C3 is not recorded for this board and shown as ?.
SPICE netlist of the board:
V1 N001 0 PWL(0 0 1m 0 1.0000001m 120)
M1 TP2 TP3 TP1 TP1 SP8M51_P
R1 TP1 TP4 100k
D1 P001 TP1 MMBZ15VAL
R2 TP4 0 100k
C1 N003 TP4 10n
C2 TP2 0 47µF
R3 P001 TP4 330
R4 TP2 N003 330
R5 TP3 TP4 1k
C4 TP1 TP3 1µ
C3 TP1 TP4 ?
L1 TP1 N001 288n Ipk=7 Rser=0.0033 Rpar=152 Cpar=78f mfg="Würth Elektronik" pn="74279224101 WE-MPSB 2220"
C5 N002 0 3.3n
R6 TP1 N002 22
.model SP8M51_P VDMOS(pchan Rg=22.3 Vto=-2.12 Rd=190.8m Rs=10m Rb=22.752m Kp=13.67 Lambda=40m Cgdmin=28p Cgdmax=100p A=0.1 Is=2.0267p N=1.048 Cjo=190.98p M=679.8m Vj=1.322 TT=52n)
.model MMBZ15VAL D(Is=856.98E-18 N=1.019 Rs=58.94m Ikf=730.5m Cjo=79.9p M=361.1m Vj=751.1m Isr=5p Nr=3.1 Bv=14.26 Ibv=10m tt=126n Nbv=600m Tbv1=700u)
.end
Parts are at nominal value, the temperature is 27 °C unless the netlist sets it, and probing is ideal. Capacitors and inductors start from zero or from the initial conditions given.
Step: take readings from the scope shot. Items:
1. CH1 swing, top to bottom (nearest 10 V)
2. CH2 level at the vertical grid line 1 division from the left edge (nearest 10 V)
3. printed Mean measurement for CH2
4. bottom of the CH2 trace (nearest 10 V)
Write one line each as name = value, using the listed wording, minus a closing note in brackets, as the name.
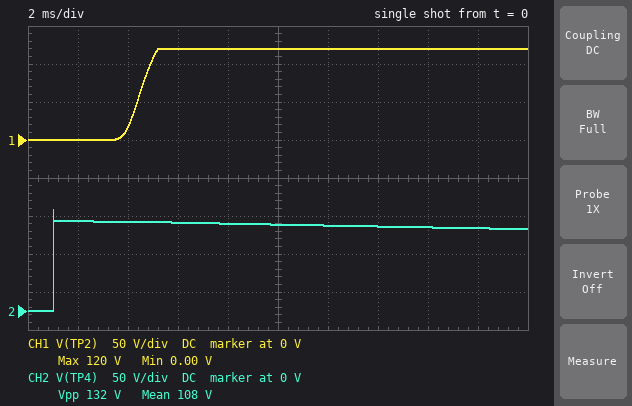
CH1 swing, top to bottom = 120 V
CH2 level at the vertical grid line 1 division from the left edge = 120 V
printed Mean measurement for CH2 = 108 V
bottom of the CH2 trace = 0 V
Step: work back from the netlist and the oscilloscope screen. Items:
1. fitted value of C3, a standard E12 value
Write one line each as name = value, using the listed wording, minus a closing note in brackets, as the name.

fitted value of C3, a standard E12 value = 680 nF
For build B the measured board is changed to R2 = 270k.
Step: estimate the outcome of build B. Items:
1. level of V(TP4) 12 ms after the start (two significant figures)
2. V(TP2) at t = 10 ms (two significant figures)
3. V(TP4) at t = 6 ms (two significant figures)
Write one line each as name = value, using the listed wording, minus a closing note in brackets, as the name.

level of V(TP4) 12 ms after the start = 120 V
V(TP2) at t = 10 ms = 83 V
V(TP4) at t = 6 ms = 120 V
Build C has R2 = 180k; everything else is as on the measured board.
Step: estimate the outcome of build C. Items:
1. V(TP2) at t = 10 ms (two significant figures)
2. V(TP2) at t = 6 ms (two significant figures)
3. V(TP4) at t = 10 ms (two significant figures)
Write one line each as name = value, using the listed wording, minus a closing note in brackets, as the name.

V(TP2) at t = 10 ms = 120 V
V(TP2) at t = 6 ms = 20 V
V(TP4) at t = 10 ms = 120 V
